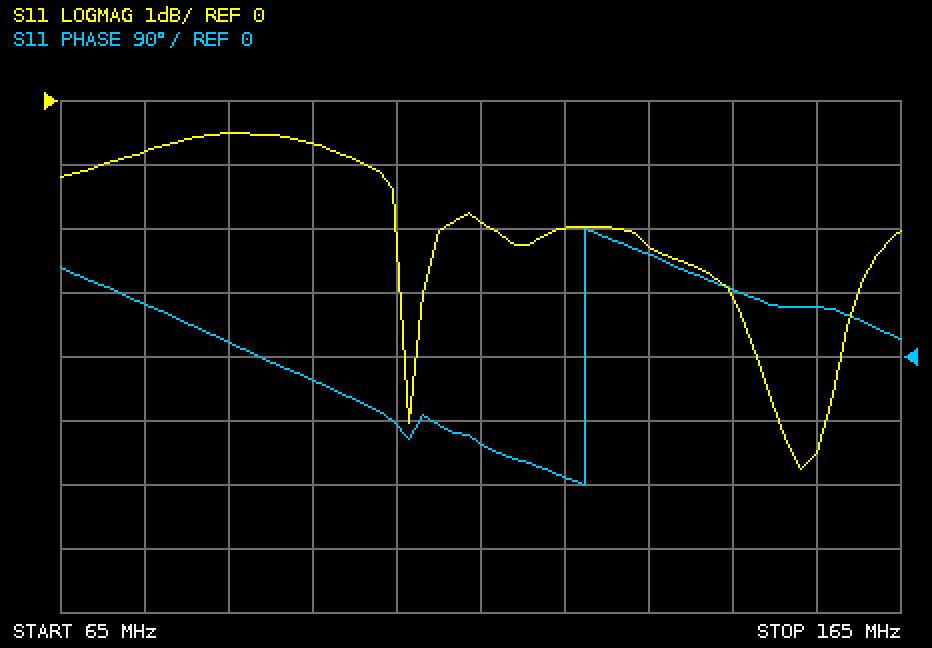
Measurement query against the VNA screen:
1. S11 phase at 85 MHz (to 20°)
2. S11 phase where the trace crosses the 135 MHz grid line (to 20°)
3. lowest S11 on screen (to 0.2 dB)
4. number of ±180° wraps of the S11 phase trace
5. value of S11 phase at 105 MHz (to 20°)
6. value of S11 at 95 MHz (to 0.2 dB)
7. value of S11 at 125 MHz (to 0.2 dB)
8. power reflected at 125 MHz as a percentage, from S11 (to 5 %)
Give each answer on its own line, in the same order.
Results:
20°
140°
-5.8 dB
1
-100°
-0.6 dB
-2.0 dB
65 %
